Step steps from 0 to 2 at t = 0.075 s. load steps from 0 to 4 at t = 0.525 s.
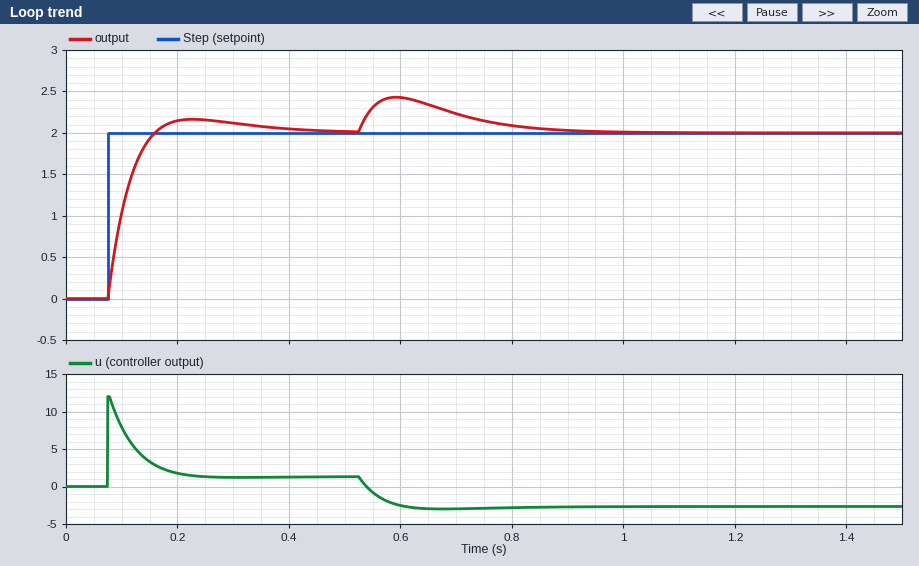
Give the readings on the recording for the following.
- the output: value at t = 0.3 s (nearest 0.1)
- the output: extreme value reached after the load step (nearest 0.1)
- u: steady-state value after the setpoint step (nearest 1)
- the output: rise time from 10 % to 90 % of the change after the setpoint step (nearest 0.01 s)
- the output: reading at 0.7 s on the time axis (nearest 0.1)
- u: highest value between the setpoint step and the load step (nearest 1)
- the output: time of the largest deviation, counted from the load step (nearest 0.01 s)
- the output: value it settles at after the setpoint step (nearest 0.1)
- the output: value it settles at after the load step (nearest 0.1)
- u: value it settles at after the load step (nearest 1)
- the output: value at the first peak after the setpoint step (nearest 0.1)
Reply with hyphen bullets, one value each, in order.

- 2.1
- 2.4
- 1
- 0.06 s
- 2.2
- 12
- 0.07 s
- 2.0
- 2.0
- -3
- 2.2
